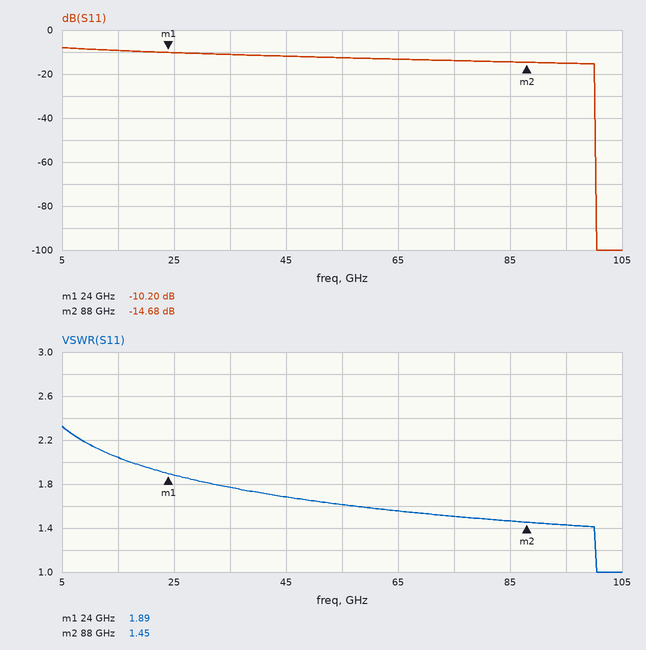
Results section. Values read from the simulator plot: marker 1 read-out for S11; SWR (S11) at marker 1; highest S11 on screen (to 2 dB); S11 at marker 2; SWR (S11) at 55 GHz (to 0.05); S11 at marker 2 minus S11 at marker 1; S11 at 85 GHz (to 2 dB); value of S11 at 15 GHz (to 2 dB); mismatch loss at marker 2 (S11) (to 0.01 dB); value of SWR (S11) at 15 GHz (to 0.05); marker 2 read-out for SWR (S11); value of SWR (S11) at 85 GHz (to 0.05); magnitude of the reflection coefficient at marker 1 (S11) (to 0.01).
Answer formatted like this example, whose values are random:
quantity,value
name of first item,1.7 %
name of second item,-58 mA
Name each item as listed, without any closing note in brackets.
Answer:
quantity,value
marker 1 read-out for S11,-10.20 dB
SWR (S11) at marker 1,1.89
highest S11 on screen,-8 dB
S11 at marker 2,-14.68 dB
SWR (S11) at 55 GHz,1.60
S11 at marker 2 minus S11 at marker 1,-4.48 dB
S11 at 85 GHz,-14 dB
value of S11 at 15 GHz,-10 dB
mismatch loss at marker 2 (S11),0.15 dB
value of SWR (S11) at 15 GHz,2.05
marker 2 read-out for SWR,1.45
value of SWR (S11) at 85 GHz,1.45
magnitude of the reflection coefficient at marker 1 (S11),0.31
